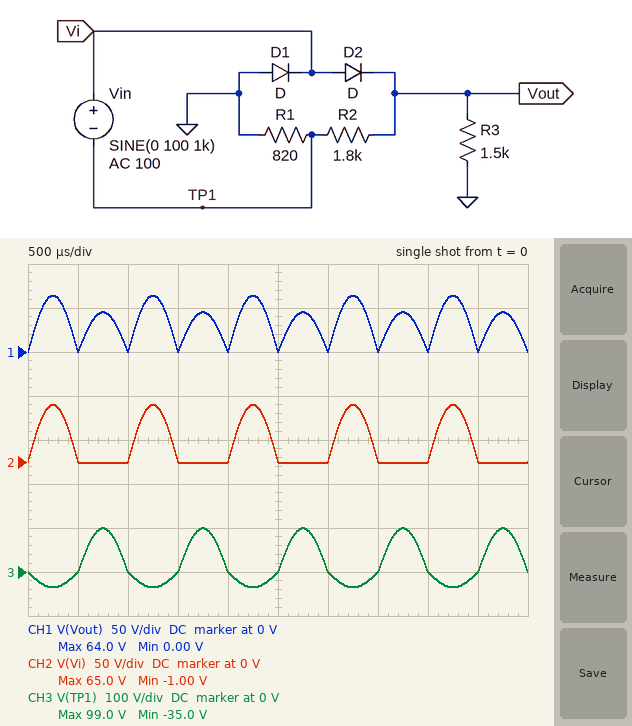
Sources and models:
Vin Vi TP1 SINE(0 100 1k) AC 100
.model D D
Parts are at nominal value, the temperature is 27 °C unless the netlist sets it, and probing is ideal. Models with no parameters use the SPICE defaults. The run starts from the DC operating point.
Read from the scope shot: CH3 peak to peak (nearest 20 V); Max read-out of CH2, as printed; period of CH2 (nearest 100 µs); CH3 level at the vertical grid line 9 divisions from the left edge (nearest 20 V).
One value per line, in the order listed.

140 V
65.0 V
1.0 ms
0 V
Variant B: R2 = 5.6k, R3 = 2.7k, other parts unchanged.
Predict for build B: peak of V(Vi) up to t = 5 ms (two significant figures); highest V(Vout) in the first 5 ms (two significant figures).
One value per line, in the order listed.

77 V
76 V
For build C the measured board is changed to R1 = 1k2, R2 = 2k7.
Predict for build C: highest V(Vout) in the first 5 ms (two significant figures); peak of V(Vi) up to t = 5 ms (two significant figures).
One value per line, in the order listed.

55 V
56 V
